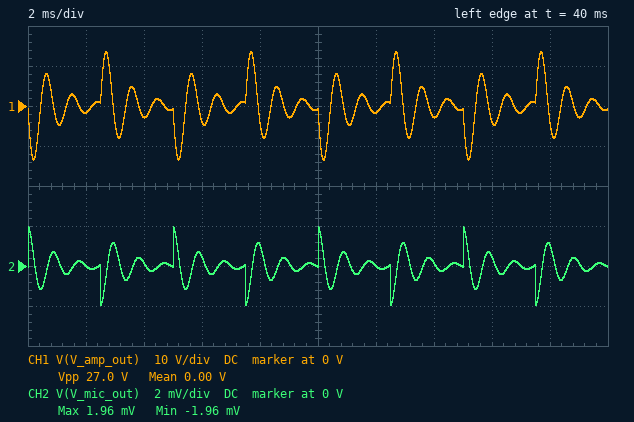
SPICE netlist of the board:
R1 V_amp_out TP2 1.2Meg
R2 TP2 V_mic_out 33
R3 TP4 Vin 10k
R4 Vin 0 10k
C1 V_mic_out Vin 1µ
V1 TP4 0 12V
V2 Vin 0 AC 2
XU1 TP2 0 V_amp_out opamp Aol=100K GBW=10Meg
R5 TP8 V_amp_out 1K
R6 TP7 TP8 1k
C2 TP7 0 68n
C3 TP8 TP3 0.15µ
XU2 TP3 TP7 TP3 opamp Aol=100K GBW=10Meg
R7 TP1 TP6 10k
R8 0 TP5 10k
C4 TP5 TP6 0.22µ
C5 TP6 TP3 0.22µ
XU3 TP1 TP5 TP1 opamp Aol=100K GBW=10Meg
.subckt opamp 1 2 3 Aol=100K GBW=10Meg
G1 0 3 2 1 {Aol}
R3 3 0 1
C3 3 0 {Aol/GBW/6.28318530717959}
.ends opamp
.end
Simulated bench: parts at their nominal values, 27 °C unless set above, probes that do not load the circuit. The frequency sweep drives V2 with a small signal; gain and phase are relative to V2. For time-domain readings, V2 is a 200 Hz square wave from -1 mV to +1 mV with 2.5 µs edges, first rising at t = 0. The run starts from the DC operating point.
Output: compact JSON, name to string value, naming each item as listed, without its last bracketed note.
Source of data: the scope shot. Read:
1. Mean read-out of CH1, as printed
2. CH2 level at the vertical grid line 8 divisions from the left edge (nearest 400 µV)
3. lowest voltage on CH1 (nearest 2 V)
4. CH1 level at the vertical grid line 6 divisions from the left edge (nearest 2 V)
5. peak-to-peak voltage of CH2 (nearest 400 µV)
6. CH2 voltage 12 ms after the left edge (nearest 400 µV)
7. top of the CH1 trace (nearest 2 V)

{"Mean read-out of CH1, as printed": "0.00 V", "CH2 level at the vertical grid line 8 divisions from the left edge": "400 µV", "lowest voltage on CH1": "-14 V", "CH1 level at the vertical grid line 6 divisions from the left edge": "-2 V", "peak-to-peak voltage of CH2": "4.0 mV", "CH2 voltage 12 ms after the left edge": "0 V", "top of the CH1 trace": "14 V"}
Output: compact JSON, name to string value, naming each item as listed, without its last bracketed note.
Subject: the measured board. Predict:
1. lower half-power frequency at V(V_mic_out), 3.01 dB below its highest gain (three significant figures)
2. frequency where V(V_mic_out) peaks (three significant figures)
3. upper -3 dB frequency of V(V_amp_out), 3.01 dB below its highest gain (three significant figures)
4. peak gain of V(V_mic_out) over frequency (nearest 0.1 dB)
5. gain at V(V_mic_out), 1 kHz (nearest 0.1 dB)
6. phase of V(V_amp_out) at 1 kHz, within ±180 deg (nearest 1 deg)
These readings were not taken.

{"lower half-power frequency at V(V_mic_out), 3.01 dB below its highest gain": "1.02 kHz", "frequency where V(V_mic_out) peaks": "1.18 kHz", "upper -3 dB frequency of V(V_amp_out), 3.01 dB below its highest gain": "1.35 kHz", "peak gain of V(V_mic_out) over frequency": "10.3 dB", "gain at V(V_mic_out), 1 kHz": "6.6 dB", "phase of V(V_amp_out) at 1 kHz, within ±180 deg": "-139 deg"}
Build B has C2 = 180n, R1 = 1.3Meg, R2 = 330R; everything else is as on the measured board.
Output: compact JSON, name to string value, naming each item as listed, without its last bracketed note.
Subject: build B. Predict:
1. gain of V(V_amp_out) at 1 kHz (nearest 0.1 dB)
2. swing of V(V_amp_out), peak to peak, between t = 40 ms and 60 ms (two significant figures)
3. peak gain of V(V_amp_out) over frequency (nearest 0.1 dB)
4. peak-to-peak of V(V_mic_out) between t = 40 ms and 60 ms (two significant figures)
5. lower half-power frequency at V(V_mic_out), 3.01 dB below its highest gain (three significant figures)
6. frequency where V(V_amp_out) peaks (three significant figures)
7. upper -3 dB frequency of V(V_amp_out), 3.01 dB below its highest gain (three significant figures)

{"gain of V(V_amp_out) at 1 kHz": "71.5 dB", "swing of V(V_amp_out), peak to peak, between t = 40 ms and 60 ms": "12 V", "peak gain of V(V_amp_out) over frequency": "71.6 dB", "peak-to-peak of V(V_mic_out) between t = 40 ms and 60 ms": "4.0 mV", "lower half-power frequency at V(V_mic_out), 3.01 dB below its highest gain": "469 Hz", "frequency where V(V_amp_out) peaks": "1.11 kHz", "upper -3 dB frequency of V(V_amp_out), 3.01 dB below its highest gain": "3.04 kHz"}
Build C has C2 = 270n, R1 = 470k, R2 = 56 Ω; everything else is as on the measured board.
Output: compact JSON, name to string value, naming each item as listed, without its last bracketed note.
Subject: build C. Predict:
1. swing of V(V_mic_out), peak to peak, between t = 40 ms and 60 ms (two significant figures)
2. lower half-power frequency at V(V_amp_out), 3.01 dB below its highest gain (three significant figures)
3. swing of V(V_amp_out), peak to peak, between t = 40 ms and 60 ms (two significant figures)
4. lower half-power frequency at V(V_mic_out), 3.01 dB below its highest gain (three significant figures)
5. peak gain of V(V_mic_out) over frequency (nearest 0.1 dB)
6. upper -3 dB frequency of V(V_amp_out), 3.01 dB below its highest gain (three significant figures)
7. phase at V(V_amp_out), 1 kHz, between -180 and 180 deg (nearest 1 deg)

{"swing of V(V_mic_out), peak to peak, between t = 40 ms and 60 ms": "4.0 mV", "lower half-power frequency at V(V_amp_out), 3.01 dB below its highest gain": "1.30 kHz", "swing of V(V_amp_out), peak to peak, between t = 40 ms and 60 ms": "14 V", "lower half-power frequency at V(V_mic_out), 3.01 dB below its highest gain": "1.47 kHz", "peak gain of V(V_mic_out) over frequency": "5.1 dB", "upper -3 dB frequency of V(V_amp_out), 3.01 dB below its highest gain": "2.60 kHz", "phase at V(V_amp_out), 1 kHz, between -180 and 180 deg": "-118 deg"}
